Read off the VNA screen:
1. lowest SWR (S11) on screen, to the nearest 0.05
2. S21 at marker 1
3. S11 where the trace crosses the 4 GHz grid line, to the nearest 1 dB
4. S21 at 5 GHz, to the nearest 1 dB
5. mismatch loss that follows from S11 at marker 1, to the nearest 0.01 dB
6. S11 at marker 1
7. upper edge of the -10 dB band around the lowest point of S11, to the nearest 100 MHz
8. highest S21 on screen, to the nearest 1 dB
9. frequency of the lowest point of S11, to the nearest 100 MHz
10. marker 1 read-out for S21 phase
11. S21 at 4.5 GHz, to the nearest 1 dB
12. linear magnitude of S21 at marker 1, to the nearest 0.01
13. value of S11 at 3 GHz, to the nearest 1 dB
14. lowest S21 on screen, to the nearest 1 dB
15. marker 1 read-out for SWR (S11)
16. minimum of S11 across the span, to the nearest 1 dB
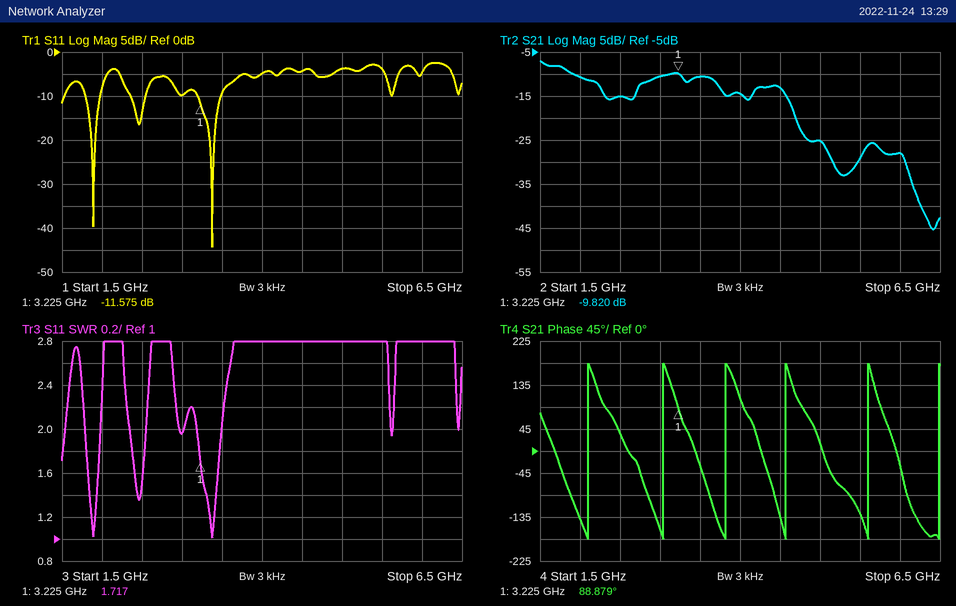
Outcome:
1.00
-9.820 dB
-5 dB
-25 dB
0.31 dB
-11.575 dB
3.5 GHz
-7 dB
3.4 GHz
88.879°
-13 dB
0.32
-10 dB
-45 dB
1.717
-44 dB
